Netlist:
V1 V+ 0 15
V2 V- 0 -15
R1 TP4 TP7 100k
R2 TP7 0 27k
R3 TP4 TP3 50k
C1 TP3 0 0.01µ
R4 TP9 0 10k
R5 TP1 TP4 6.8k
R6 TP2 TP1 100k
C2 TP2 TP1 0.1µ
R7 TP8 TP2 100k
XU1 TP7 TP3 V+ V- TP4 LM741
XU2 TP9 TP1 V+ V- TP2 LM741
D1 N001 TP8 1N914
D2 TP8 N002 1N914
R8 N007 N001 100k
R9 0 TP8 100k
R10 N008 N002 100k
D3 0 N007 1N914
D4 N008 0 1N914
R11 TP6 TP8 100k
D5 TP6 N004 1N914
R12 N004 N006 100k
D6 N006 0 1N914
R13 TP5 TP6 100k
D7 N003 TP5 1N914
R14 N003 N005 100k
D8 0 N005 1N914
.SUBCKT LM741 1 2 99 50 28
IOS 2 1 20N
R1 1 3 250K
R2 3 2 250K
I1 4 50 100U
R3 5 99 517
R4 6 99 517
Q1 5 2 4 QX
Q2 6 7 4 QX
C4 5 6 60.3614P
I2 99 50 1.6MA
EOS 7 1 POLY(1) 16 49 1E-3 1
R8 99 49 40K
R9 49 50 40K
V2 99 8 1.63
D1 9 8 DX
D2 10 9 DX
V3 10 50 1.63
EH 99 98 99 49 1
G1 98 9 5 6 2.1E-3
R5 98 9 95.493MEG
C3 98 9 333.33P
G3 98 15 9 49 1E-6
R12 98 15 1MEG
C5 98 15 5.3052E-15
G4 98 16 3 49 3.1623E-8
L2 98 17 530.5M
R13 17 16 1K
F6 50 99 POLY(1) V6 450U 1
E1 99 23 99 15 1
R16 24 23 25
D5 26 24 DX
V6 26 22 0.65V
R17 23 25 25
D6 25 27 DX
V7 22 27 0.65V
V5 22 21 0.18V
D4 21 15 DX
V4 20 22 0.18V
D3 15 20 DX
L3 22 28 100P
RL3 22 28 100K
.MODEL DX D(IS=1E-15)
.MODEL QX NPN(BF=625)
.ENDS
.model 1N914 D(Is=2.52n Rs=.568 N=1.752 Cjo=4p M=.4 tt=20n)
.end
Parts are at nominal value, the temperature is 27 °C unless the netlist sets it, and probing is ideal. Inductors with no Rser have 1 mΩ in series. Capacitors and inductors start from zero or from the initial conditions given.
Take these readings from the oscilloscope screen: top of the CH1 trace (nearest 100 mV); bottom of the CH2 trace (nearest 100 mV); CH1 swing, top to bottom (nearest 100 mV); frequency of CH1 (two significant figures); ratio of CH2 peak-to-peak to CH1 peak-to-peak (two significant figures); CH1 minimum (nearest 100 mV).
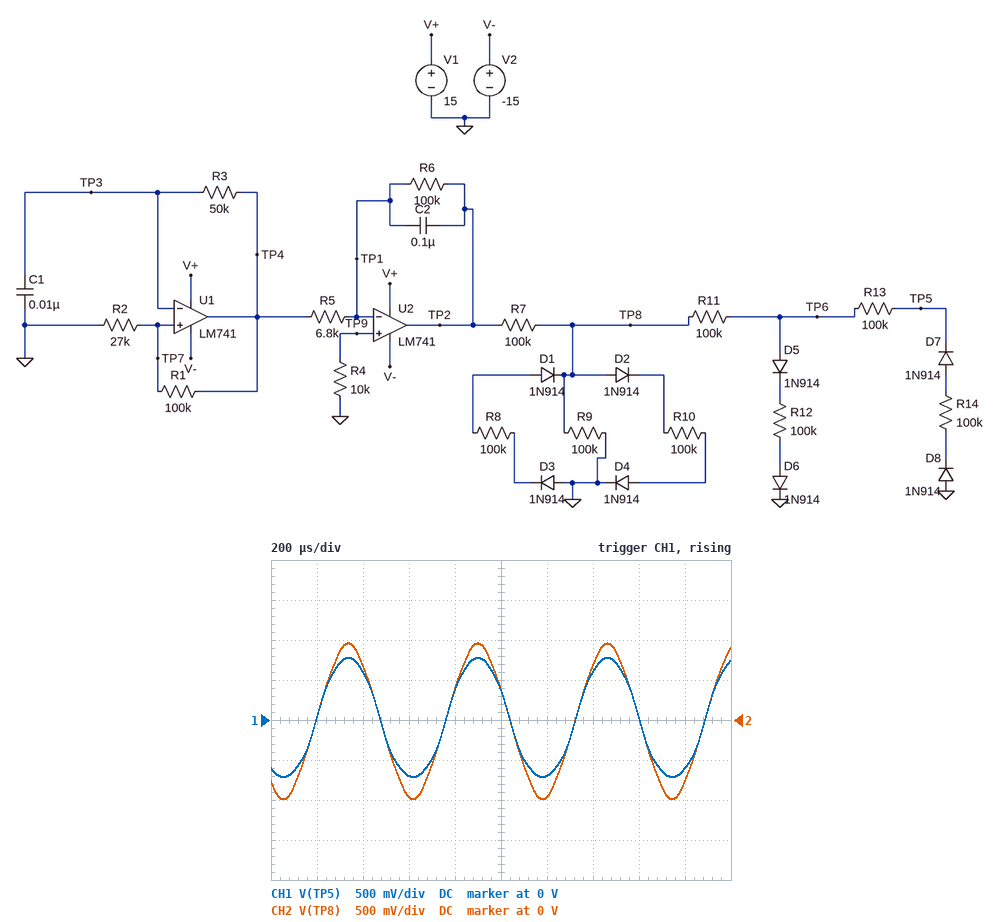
800 mV
-1.0 V
1.5 V
1.8 kHz
1.3
-700 mV
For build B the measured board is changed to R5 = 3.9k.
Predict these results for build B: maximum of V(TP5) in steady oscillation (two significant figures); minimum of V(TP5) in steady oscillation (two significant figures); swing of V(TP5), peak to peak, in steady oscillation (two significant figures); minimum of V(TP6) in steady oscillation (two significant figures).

1.1 V
-950 mV
2.0 V
-1.3 V
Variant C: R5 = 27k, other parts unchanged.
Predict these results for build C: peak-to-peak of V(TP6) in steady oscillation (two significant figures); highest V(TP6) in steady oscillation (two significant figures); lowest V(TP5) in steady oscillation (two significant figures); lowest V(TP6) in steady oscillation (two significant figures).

590 mV
300 mV
-290 mV
-300 mV
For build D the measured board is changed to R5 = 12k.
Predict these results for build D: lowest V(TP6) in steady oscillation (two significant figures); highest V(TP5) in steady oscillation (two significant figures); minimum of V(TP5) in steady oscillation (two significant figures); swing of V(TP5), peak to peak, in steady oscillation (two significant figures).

-580 mV
550 mV
-530 mV
1.1 V
